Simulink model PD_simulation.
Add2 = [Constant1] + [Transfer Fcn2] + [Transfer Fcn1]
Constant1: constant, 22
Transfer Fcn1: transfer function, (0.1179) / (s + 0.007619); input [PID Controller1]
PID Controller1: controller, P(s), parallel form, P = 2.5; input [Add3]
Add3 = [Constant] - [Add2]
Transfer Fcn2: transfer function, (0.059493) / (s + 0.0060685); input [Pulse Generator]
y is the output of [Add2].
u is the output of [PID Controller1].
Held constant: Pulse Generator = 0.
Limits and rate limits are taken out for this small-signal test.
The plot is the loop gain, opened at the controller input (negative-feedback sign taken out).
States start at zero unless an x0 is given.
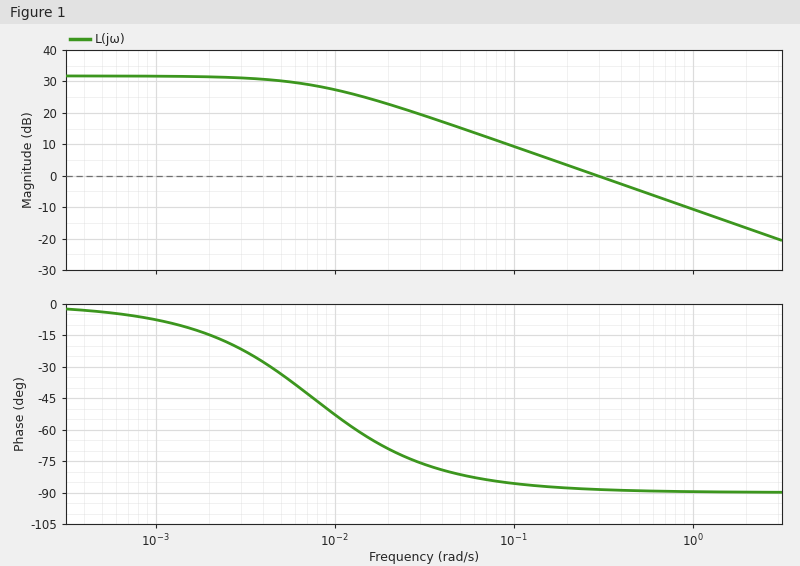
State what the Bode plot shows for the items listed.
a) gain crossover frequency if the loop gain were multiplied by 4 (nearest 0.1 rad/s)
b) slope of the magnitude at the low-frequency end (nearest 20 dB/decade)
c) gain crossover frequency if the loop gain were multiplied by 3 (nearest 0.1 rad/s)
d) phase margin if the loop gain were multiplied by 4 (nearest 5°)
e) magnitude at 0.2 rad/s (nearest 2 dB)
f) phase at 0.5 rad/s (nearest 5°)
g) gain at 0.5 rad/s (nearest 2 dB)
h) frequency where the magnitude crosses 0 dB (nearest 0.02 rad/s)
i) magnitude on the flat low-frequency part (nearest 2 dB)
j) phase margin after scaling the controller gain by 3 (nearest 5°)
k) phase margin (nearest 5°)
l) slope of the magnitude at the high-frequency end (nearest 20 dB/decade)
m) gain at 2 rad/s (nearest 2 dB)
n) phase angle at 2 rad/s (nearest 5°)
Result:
1.2 rad/s
0 dB/decade
0.9 rad/s
90°
4 dB
-90°
-4 dB
0.30 rad/s
32 dB
90°
90°
-20 dB/decade
-16 dB
-90°
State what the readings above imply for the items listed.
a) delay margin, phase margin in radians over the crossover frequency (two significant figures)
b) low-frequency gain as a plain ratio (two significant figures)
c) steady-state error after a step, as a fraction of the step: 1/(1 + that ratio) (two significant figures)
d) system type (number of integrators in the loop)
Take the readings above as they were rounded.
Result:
5.2 s
40
0.024
0
